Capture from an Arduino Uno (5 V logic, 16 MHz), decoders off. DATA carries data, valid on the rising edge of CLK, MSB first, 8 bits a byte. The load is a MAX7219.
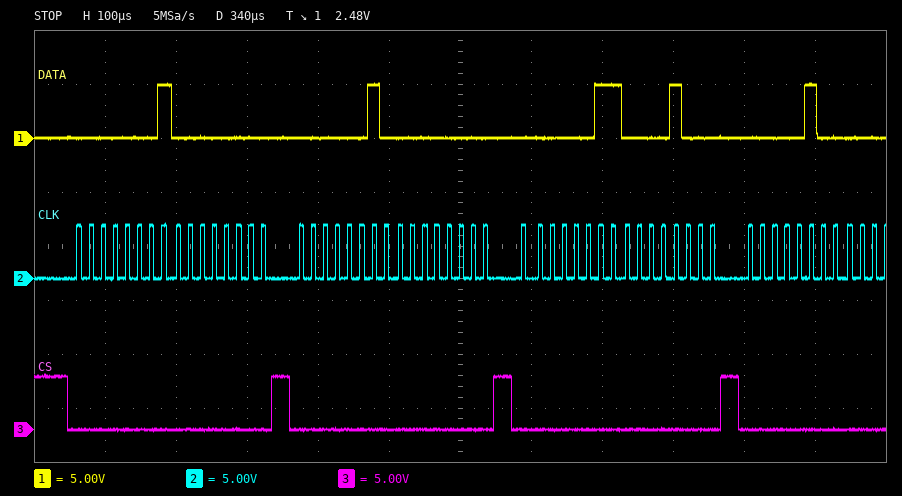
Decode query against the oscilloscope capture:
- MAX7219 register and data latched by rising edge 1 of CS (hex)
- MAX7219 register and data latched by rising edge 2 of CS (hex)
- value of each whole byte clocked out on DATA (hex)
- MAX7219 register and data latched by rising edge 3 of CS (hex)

register 0x1, data 0x00
register 0x2, data 0x00
01 00 02 00 03 08 04
register 0x3, data 0x08
